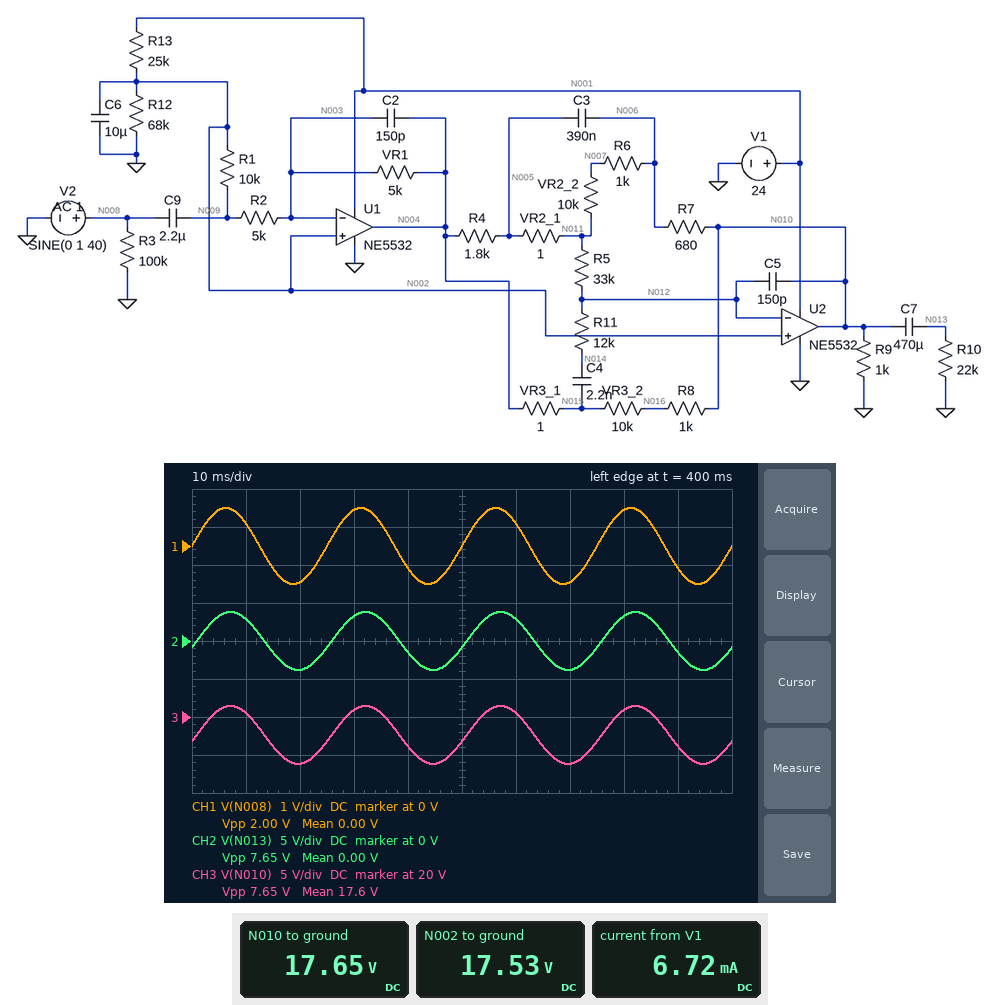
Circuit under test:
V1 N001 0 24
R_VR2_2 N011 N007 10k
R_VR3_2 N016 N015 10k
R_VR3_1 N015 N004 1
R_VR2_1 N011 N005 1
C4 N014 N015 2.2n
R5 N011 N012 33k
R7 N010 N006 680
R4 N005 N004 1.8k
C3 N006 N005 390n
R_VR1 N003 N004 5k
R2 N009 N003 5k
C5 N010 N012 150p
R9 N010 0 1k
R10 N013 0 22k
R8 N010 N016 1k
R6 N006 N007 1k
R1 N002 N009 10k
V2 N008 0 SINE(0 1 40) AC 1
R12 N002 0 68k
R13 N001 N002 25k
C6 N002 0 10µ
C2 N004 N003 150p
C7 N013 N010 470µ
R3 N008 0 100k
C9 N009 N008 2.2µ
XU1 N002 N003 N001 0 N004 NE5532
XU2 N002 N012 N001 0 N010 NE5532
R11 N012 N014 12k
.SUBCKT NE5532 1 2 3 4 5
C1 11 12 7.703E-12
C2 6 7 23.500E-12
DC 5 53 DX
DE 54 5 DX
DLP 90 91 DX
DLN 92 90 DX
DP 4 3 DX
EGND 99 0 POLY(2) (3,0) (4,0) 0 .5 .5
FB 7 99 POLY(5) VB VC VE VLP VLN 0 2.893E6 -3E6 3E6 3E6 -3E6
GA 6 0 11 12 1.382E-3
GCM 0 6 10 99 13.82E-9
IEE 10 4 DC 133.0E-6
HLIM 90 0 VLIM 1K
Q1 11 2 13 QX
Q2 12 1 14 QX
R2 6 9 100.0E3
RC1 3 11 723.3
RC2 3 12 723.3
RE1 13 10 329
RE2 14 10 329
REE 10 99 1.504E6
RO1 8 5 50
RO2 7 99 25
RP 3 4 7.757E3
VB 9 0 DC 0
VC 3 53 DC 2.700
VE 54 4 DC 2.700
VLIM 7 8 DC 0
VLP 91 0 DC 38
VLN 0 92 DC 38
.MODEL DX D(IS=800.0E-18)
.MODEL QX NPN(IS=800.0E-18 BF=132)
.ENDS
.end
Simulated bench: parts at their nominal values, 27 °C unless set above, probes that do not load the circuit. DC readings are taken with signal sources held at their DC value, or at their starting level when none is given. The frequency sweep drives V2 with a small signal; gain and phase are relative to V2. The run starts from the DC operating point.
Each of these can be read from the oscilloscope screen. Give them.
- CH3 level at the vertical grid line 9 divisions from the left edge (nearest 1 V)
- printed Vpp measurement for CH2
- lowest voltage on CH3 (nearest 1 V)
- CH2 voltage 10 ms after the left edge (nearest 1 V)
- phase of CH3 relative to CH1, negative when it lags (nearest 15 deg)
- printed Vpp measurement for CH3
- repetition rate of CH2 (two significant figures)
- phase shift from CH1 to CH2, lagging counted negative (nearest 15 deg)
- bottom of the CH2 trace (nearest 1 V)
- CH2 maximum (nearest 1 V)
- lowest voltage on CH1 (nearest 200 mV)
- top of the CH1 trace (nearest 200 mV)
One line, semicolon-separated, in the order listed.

16 V; 7.65 V; 14 V; 3 V; -15 deg; 7.65 V; 40 Hz; -15 deg; -4 V; 4 V; -1.0 V; 1.0 V
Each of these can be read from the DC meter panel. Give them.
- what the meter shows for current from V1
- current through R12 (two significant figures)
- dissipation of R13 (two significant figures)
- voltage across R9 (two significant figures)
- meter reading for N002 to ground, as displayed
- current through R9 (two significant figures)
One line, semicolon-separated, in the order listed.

6.72 mA; 260 µA; 1.7 mW; 18 V; 17.53 V; 18 mA
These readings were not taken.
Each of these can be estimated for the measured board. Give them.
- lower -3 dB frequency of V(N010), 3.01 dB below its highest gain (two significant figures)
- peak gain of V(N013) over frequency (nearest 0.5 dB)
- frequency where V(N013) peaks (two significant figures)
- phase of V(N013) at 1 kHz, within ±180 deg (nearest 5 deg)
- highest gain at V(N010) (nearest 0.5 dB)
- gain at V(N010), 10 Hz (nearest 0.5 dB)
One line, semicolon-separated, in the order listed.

12 Hz; 12.0 dB; 29 Hz; 30 deg; 12.0 dB; 8.0 dB
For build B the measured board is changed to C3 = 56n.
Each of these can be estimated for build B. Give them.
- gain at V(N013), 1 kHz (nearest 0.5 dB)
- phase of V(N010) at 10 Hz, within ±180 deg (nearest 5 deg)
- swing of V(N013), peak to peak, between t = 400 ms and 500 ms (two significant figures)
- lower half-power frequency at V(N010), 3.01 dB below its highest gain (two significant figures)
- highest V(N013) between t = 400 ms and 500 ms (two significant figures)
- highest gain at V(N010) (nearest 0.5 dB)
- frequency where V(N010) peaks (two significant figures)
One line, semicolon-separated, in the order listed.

4.5 dB; 65 deg; 9.9 V; 20 Hz; 4.3 V; 15.5 dB; 76 Hz
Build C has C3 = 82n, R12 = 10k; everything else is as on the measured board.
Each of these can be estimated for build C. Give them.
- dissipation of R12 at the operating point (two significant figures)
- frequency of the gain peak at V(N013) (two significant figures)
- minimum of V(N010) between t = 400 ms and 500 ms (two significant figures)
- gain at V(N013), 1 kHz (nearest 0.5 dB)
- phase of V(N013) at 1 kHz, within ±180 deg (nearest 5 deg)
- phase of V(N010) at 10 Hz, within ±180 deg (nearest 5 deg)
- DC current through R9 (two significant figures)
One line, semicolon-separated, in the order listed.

4.7 mW; 63 Hz; 2.0 V; 1.5 dB; -20 deg; 60 deg; 7.0 mA
